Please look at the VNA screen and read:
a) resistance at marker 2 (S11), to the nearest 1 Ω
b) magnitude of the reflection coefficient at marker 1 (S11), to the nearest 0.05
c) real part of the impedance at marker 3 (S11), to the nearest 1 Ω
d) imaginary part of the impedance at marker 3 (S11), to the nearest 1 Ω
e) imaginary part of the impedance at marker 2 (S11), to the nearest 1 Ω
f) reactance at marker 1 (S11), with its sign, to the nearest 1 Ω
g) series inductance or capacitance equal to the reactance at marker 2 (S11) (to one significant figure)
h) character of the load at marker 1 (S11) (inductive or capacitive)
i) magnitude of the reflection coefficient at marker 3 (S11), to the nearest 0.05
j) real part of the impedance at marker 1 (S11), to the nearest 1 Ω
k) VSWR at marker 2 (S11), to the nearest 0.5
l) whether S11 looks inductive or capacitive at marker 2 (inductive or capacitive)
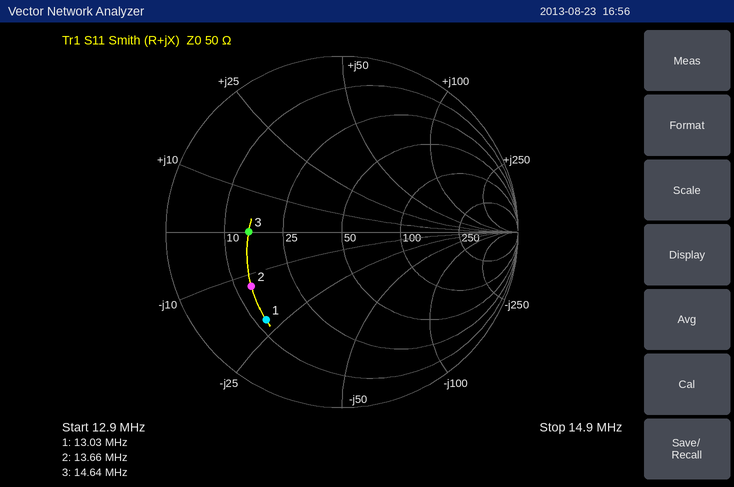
13 Ω
0.65
15 Ω
0 Ω
-13 Ω
-22 Ω
900 pF
capacitive
0.55
12 Ω
4.0
capacitive
